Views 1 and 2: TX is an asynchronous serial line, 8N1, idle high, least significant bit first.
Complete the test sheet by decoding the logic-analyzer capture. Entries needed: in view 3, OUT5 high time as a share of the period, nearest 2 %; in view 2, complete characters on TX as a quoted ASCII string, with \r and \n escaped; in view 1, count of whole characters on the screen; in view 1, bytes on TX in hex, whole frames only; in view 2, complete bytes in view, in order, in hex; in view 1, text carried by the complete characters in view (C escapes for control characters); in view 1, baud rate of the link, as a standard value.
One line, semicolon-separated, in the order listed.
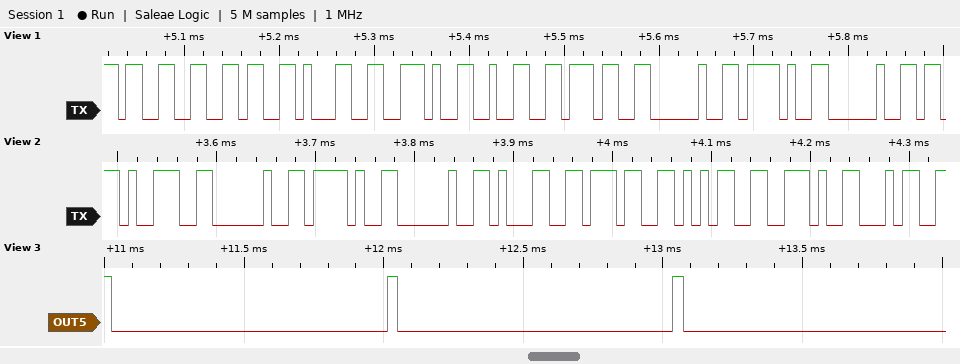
4 %; "9 / 175.4"; 9; 33 36 31 2E 32 37 20 2F 20; 39 20 2F 20 31 37 35 2E 34; "361.27 / "; 115200 baud
